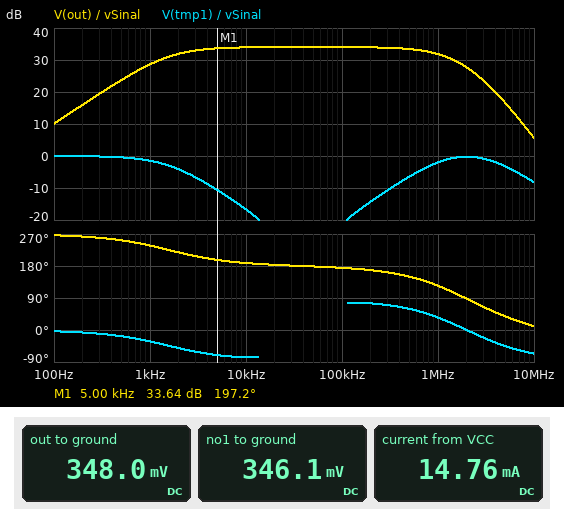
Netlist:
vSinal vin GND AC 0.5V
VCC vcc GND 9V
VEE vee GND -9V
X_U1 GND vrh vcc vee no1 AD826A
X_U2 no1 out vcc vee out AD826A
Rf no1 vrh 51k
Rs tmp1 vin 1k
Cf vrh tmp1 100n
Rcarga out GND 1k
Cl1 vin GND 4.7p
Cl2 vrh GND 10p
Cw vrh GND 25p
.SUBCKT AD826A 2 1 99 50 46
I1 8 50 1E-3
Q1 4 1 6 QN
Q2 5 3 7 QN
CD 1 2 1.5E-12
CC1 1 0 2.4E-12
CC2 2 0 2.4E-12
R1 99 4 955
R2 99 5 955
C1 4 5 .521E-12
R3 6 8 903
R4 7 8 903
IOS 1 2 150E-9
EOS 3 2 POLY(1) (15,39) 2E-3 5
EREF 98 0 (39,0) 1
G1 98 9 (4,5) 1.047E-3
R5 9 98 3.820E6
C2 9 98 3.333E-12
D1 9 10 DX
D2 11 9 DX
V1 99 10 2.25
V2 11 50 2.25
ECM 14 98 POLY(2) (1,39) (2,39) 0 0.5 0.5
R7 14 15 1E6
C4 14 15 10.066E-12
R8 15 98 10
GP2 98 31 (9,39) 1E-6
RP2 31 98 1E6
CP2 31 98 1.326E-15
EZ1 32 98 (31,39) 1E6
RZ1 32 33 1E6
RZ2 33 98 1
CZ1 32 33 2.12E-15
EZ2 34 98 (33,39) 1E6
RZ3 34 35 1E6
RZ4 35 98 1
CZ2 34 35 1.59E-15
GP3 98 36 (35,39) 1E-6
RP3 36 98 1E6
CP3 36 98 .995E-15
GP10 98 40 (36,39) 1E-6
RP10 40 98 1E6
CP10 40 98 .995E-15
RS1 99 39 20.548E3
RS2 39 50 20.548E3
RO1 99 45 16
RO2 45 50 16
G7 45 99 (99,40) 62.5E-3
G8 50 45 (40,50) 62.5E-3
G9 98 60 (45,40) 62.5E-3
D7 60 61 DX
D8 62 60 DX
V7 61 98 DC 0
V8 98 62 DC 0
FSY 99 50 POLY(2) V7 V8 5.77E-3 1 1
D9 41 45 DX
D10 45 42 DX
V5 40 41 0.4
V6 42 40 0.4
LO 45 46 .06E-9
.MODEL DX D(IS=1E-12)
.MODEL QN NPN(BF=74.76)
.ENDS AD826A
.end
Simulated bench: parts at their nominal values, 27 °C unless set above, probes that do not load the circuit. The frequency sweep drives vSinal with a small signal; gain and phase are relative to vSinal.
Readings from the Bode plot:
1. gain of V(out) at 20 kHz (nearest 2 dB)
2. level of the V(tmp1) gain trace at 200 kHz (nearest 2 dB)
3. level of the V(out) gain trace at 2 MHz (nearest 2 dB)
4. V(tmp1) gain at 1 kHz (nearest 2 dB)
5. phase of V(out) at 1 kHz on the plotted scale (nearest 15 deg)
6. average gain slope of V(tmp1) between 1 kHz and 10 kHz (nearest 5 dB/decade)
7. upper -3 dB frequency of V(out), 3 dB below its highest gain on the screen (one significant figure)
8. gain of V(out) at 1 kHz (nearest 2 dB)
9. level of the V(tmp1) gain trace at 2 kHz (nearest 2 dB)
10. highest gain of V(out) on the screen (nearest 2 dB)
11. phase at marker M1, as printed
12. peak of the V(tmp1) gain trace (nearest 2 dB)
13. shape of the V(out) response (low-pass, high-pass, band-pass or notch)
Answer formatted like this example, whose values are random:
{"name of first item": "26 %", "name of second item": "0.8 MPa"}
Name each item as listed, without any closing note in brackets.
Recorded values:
{"gain of V(out) at 20 kHz": "34 dB", "level of the V(tmp1) gain trace at 200 kHz": "-14 dB", "level of the V(out) gain trace at 2 MHz": "28 dB", "V(tmp1) gain at 1 kHz": "-2 dB", "phase of V(out) at 1 kHz on the plotted scale": "240 deg", "average gain slope of V(tmp1) between 1 kHz and 10 kHz": "-15 dB/decade", "upper -3 dB frequency of V(out), 3 dB below its highest gain on the screen": "1 MHz", "gain of V(out) at 1 kHz": "28 dB", "level of the V(tmp1) gain trace at 2 kHz": "-4 dB", "highest gain of V(out) on the screen": "34 dB", "phase at marker M1, as printed": "197.2 deg", "peak of the V(tmp1) gain trace": "0 dB", "shape of the V(out) response": "band-pass"}
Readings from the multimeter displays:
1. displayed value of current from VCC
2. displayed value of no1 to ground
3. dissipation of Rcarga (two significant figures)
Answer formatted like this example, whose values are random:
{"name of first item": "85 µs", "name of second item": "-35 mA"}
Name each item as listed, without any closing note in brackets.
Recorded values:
{"displayed value of current from VCC": "14.76 mA", "displayed value of no1 to ground": "346.1 mV", "dissipation of Rcarga": "120 µW"}
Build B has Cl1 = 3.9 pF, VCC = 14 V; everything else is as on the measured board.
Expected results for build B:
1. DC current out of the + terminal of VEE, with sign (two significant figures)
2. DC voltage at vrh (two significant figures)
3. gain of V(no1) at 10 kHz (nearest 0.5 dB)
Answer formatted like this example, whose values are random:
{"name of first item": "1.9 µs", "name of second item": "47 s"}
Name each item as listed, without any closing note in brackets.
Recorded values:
{"DC current out of the + terminal of VEE, with sign": "-15 mA", "DC voltage at vrh": "2.4 mV", "gain of V(no1) at 10 kHz": "34.0 dB"}
